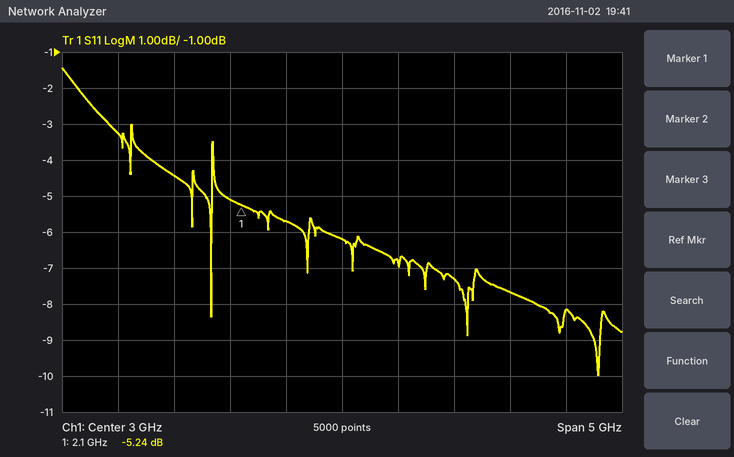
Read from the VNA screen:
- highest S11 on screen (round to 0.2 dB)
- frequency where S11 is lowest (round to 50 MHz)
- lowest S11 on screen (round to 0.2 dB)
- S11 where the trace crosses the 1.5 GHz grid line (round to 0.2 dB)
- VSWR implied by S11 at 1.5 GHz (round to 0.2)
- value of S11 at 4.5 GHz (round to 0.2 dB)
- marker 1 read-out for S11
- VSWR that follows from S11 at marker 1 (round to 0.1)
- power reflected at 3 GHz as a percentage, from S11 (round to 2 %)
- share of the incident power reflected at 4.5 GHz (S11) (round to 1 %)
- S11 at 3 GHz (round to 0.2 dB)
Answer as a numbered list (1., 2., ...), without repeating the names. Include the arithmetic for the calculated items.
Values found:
1. -1.4 dB
2. 5.30 GHz
3. -10.0 dB
4. -4.4 dB
5. |Γ| = 10^(-4.4/20) = 0.6026; VSWR = (1 + 0.6026)/(1 − 0.6026) ≈ 4.0
6. -7.6 dB
7. -5.24 dB
8. (1 + 0.5470)/(1 − 0.5470) ≈ 3.4
9. 10^(-6.2/10) ≈ 24 %
10. 10^(-7.6/10) ≈ 17 %
11. -6.2 dB
